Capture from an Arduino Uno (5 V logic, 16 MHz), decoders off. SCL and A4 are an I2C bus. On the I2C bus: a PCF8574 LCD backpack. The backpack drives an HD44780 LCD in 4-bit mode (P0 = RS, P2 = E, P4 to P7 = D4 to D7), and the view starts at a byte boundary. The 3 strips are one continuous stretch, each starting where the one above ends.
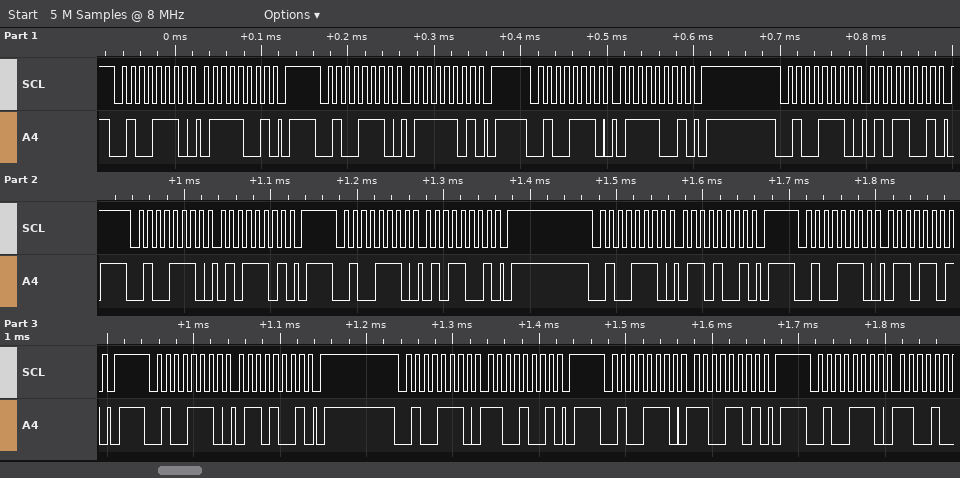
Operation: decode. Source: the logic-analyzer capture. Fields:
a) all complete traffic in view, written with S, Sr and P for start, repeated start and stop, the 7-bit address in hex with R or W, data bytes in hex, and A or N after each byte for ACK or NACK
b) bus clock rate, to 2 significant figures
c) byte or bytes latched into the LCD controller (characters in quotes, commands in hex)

S 27W A 79 A P S 27W A 7D A P S 27W A 79 A P S 27W A 59 A P S 27W A 5D A P S 27W A 59 A P S 27W A 69 A P S 27W A 6D A P S 27W A 69 A P S 27W A C9 A P S 27W A CD A P S 27W A
100 kHz
'u'
